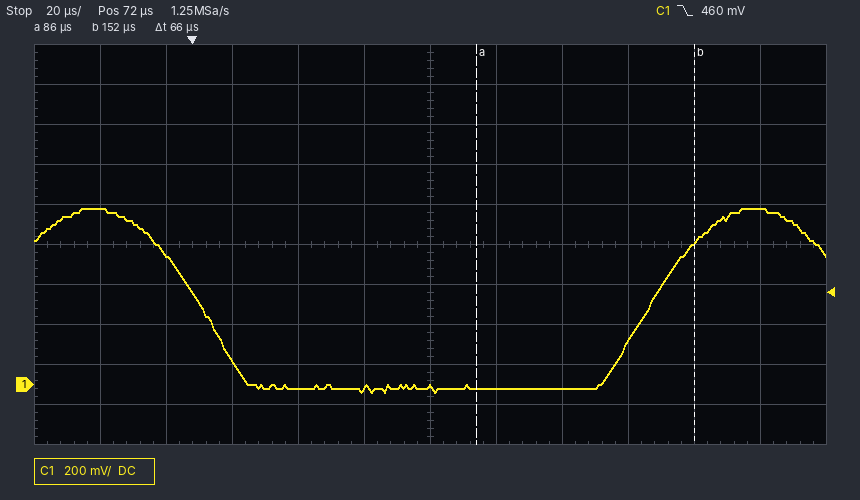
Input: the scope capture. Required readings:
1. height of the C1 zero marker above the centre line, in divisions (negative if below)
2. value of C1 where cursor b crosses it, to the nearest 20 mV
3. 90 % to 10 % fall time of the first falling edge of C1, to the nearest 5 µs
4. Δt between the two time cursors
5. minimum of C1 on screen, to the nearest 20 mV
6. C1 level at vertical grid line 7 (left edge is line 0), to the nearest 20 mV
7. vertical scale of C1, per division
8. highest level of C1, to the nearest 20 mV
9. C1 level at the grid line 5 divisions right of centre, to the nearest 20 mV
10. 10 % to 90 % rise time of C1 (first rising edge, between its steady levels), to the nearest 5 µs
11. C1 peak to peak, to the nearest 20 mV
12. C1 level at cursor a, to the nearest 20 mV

-3.5 div
720 mV
30 µs
66 µs
-40 mV
-20 mV
200 mV
880 mV
880 mV
30 µs
920 mV
-20 mV
